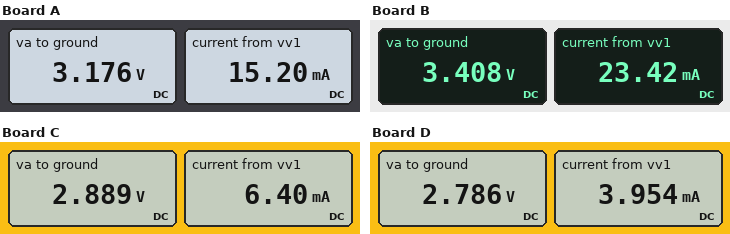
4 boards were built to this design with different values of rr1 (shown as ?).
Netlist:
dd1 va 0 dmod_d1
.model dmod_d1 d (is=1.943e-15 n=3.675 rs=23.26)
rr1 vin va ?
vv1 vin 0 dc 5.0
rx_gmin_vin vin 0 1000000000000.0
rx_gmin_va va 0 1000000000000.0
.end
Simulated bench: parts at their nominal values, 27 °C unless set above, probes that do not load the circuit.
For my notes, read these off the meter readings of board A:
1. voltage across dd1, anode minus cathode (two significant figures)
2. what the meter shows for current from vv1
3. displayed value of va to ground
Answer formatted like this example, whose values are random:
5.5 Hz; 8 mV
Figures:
3.2 V; 15.20 mA; 3.176 V
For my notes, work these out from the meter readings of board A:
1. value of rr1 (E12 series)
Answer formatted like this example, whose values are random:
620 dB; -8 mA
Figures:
120 Ω
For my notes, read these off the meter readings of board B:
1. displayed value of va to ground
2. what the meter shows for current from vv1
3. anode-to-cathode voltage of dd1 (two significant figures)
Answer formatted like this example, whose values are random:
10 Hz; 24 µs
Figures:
3.408 V; 23.42 mA; 3.4 V
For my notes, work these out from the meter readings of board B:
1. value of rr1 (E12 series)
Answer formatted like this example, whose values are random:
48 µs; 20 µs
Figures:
68 Ω
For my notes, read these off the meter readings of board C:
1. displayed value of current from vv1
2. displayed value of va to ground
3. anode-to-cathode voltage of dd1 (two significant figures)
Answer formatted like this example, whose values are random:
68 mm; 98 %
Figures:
6.40 mA; 2.889 V; 2.9 V
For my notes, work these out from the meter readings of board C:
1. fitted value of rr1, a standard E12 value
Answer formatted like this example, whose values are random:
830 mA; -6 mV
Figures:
330 Ω
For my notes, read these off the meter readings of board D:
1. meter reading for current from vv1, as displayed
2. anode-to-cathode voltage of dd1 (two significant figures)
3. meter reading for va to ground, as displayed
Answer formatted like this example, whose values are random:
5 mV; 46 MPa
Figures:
3.954 mA; 2.8 V; 2.786 V
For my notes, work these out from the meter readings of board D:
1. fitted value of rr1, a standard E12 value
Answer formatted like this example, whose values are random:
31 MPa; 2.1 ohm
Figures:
560 Ω
